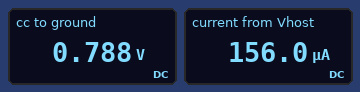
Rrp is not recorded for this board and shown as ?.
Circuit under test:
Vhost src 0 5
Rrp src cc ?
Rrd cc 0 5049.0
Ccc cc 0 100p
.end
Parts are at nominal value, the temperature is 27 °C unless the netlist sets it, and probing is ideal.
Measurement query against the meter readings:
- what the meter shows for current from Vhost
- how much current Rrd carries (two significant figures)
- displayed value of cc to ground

156.0 µA
160 µA
0.788 V
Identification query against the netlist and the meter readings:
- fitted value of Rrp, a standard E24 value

27 kΩ
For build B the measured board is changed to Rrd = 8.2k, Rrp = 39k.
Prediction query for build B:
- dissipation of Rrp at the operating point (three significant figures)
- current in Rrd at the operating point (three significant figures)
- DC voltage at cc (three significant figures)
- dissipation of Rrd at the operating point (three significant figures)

438 µW
106 µA
869 mV
92.0 µW
